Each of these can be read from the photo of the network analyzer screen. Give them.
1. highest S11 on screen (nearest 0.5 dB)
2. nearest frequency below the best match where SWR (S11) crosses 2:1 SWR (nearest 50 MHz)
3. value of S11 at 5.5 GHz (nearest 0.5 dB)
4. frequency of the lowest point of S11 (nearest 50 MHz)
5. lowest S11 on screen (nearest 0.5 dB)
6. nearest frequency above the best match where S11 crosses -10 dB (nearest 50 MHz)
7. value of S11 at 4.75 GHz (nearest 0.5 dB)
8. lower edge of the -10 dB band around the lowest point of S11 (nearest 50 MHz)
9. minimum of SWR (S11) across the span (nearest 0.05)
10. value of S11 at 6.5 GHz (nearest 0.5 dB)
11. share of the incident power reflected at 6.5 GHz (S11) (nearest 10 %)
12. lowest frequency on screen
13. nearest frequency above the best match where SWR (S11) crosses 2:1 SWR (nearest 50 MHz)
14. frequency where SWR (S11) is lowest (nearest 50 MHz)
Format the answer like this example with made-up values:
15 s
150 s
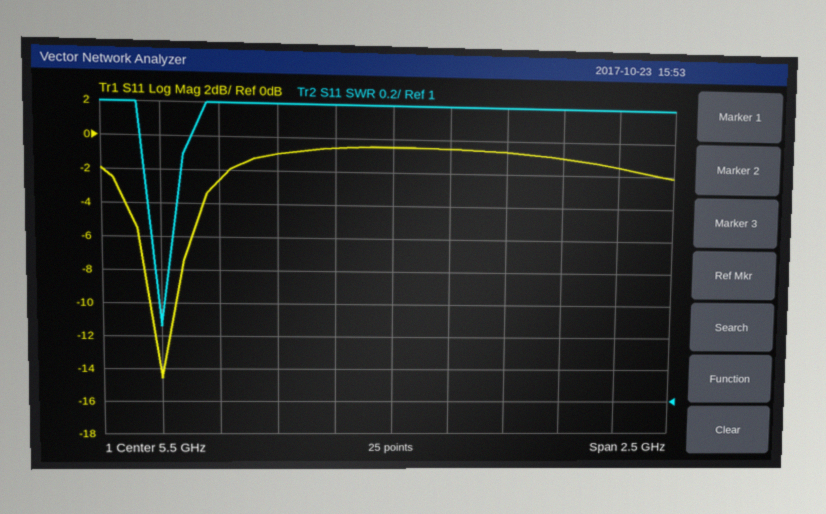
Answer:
-0.5 dB
4.45 GHz
-0.5 dB
4.50 GHz
-14.5 dB
4.55 GHz
-2.5 dB
4.45 GHz
1.45
-1.5 dB
70 %
4.25 GHz
4.55 GHz
4.50 GHz
